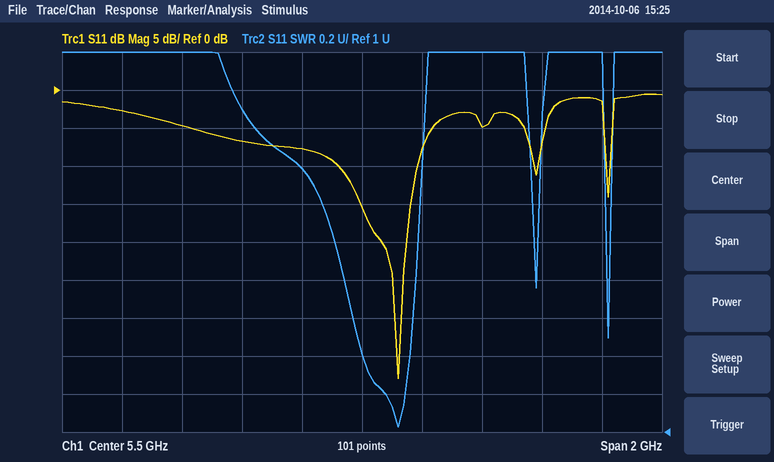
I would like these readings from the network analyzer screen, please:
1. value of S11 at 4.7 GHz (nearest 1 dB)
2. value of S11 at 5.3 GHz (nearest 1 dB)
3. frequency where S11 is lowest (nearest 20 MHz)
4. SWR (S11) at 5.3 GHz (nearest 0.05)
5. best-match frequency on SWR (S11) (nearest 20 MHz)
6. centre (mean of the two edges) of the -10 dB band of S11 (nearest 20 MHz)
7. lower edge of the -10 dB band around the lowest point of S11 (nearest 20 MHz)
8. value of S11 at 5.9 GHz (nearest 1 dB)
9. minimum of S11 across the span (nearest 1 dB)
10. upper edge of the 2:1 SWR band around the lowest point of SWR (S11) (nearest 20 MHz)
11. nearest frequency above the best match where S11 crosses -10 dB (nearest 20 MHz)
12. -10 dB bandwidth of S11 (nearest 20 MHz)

-3 dB
-8 dB
5.62 GHz
2.40
5.62 GHz
5.56 GHz
5.42 GHz
-5 dB
-38 dB
5.68 GHz
5.68 GHz
260 MHz
